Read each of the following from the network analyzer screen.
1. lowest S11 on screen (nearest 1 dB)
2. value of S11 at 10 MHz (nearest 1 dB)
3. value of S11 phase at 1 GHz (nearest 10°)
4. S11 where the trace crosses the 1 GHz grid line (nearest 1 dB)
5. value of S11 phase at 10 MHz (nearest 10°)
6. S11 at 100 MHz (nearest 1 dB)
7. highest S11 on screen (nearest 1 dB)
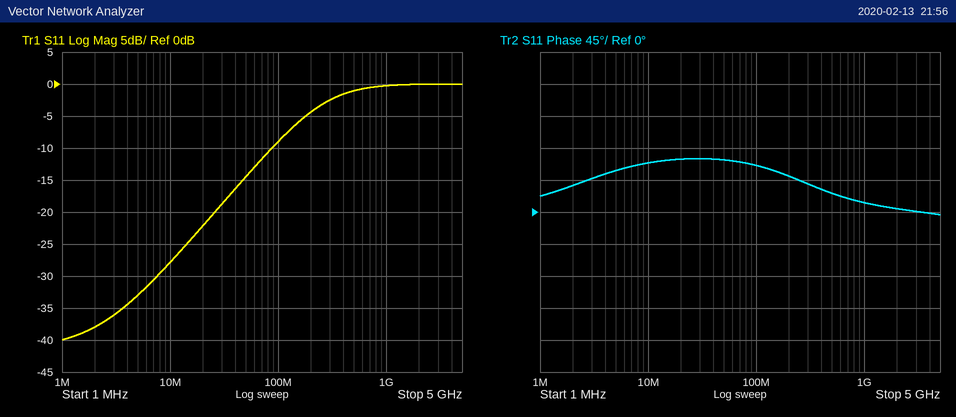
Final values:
-40 dB
-28 dB
10°
0 dB
70°
-9 dB
0 dB
